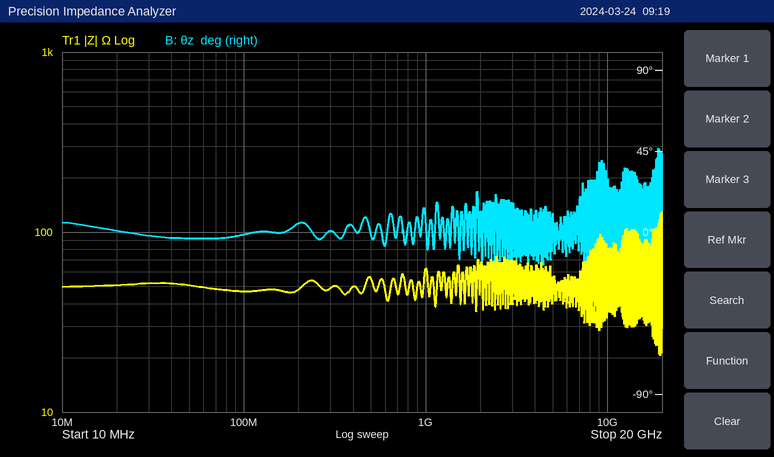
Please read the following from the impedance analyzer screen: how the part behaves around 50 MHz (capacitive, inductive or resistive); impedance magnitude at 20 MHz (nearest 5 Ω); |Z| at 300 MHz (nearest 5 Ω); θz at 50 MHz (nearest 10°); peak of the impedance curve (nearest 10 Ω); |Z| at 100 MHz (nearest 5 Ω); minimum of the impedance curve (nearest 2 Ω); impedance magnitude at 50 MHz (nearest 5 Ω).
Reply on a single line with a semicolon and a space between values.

resistive; 50 Ω; 50 Ω; 0°; 130 Ω; 45 Ω; 20 Ω; 50 Ω
